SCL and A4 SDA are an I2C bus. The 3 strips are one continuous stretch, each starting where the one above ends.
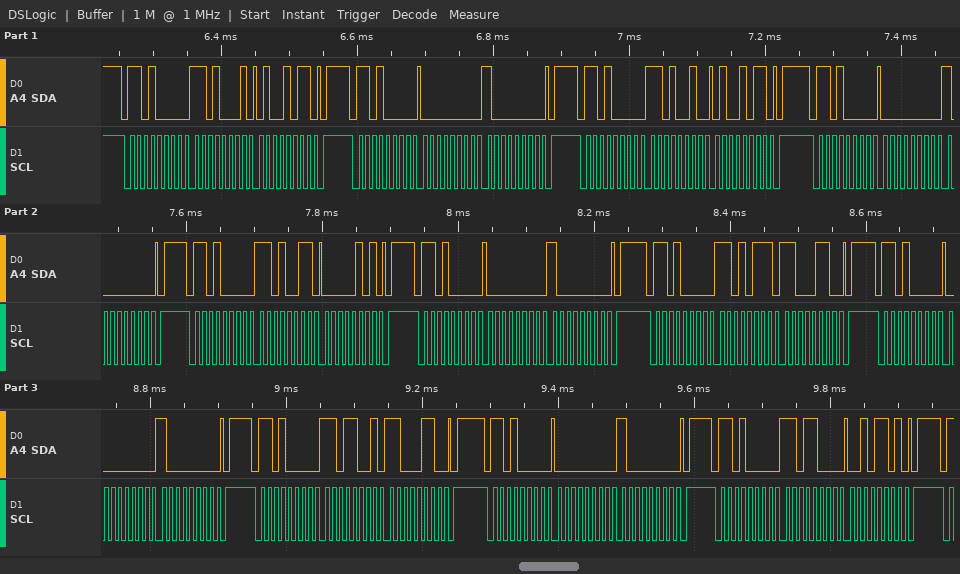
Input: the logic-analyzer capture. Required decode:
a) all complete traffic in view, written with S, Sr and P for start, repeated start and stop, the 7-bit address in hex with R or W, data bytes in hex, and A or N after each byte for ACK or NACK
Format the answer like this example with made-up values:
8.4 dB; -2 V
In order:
S 68W A D1 A 4B A P S 68W A 00 A 80 A P S 68W A D2 A 4B A P S 68W A 00 A 80 A P S 68W A D3 A 05 A P S 68W A 00 A 80 A P S 68W A D7 A C6 A P S 68W A 00 A 80 A P S 68W A D9 A C6 A P S 68W A 00 A 80 A P S 68W A D8 A 2D A P
